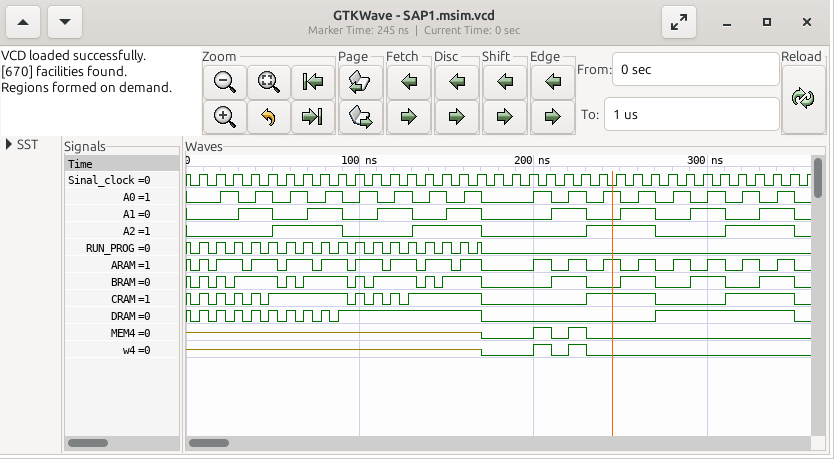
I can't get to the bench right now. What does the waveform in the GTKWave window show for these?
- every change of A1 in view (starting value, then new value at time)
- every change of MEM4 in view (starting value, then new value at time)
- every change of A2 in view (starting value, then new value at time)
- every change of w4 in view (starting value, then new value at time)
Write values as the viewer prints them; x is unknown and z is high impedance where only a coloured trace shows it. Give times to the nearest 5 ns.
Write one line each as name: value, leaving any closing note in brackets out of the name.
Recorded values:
every change of A1 in view: 0, 1 at 30 ns, 0 at 50 ns, 1 at 70 ns, 0 at 90 ns, 1 at 110 ns, 0 at 130 ns, 1 at 150 ns, 0 at 170 ns, 1 at 210 ns, 0 at 230 ns, 1 at 250 ns, 0 at 270 ns, 1 at 290 ns, 0 at 310 ns, 1 at 330 ns, 0 at 350 ns
every change of MEM4 in view: z, 0 at 170 ns, 1 at 200 ns, 0 at 210 ns, 1 at 220 ns, 0 at 230 ns
every change of A2 in view: 0, 1 at 50 ns, 0 at 90 ns, 1 at 130 ns, 0 at 170 ns, 1 at 230 ns, 0 at 270 ns, 1 at 310 ns, 0 at 350 ns
every change of w4 in view: z, 0 at 170 ns, 1 at 200 ns, 0 at 210 ns, 1 at 220 ns, 0 at 230 ns
